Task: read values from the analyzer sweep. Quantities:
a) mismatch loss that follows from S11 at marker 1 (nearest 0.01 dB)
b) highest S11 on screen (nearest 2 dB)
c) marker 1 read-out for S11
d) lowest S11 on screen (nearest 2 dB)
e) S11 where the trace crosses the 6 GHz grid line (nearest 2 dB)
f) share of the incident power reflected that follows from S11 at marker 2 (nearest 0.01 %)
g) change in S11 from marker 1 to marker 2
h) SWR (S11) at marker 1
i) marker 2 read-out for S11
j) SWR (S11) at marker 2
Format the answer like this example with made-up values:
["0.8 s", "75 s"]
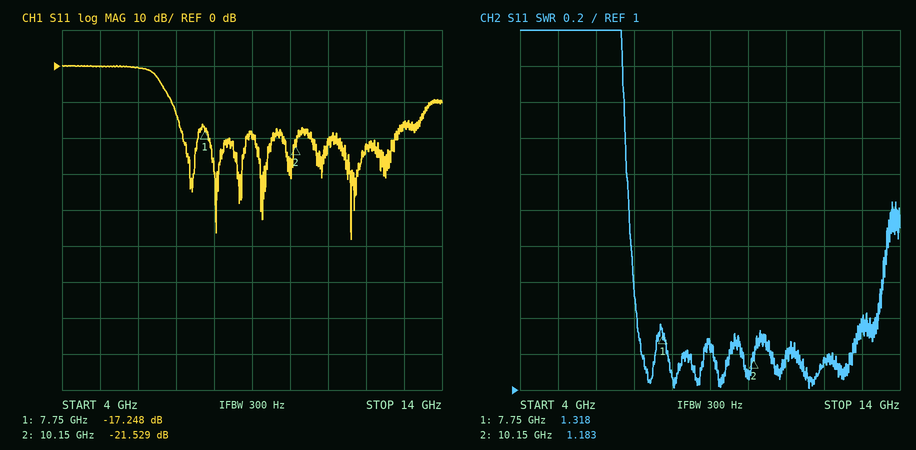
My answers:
["0.08 dB", "0 dB", "-17.248 dB", "-48 dB", "0 dB", "0.70 %", "-4.281 dB", "1.318", "-21.529 dB", "1.183"]
